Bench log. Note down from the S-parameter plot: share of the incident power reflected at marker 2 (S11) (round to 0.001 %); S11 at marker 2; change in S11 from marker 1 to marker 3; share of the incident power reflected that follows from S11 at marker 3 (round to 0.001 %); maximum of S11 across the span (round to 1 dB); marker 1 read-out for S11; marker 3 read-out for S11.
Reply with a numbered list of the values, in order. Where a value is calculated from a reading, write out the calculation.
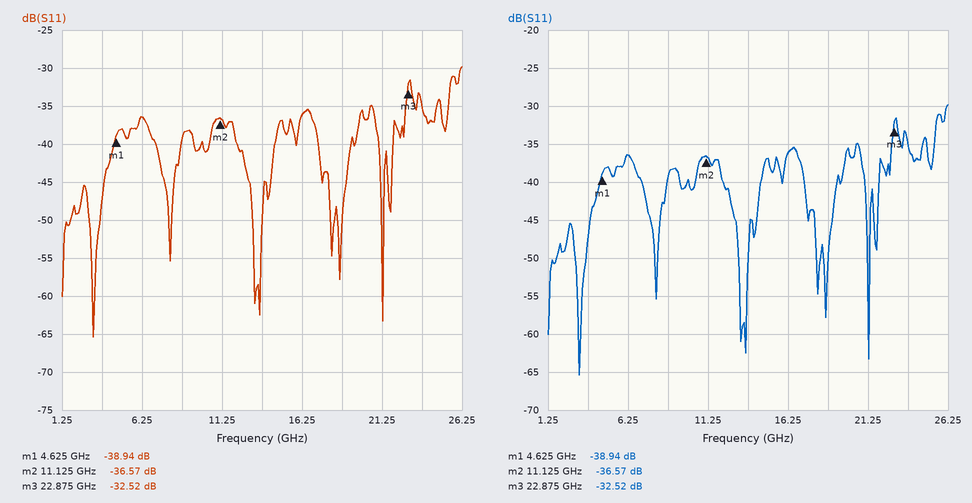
1. 10^(-36.57/10) ≈ 0.022 %
2. -36.57 dB
3. -32.52 − (-38.94) = 6.42 dB
4. 10^(-32.52/10) ≈ 0.056 %
5. -30 dB
6. -38.94 dB
7. -32.52 dB
